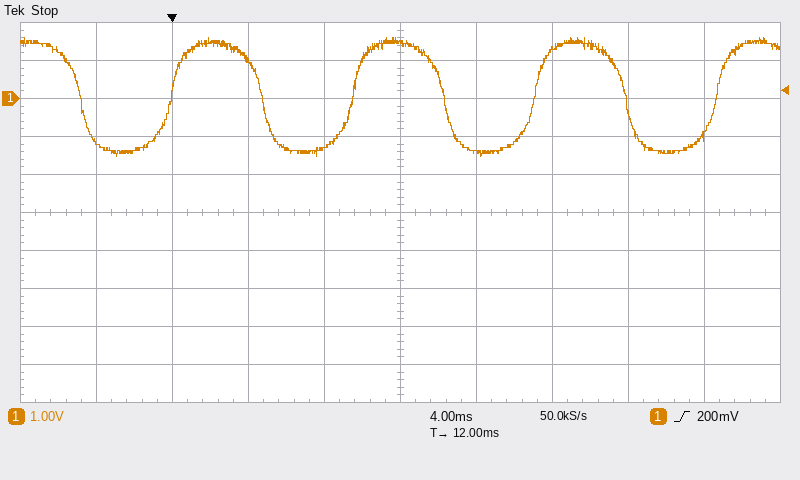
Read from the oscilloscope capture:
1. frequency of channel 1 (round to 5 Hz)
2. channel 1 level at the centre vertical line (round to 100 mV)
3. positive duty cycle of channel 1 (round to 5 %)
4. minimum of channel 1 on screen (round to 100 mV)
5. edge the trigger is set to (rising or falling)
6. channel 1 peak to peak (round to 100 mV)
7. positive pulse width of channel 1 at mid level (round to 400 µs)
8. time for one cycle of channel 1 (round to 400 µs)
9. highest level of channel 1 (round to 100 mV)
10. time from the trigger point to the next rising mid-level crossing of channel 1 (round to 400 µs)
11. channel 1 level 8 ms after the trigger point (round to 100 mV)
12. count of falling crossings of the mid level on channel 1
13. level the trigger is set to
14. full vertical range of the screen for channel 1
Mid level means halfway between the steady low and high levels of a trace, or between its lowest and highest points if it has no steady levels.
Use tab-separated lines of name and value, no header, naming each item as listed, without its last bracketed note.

frequency of channel 1	105 Hz
channel 1 level at the centre vertical line	1.4 V
positive duty cycle of channel 1	50 %
minimum of channel 1 on screen	-1.5 V
edge the trigger is set to	rising
channel 1 peak to peak	3.1 V
positive pulse width of channel 1 at mid level	4.8 ms
time for one cycle of channel 1	9.6 ms
highest level of channel 1	1.6 V
time from the trigger point to the next rising mid-level crossing of channel 1	9.6 ms
channel 1 level 8 ms after the trigger point	-1.3 V
count of falling crossings of the mid level on channel 1	4
level the trigger is set to	200 mV
full vertical range of the screen for channel 1	10 V
